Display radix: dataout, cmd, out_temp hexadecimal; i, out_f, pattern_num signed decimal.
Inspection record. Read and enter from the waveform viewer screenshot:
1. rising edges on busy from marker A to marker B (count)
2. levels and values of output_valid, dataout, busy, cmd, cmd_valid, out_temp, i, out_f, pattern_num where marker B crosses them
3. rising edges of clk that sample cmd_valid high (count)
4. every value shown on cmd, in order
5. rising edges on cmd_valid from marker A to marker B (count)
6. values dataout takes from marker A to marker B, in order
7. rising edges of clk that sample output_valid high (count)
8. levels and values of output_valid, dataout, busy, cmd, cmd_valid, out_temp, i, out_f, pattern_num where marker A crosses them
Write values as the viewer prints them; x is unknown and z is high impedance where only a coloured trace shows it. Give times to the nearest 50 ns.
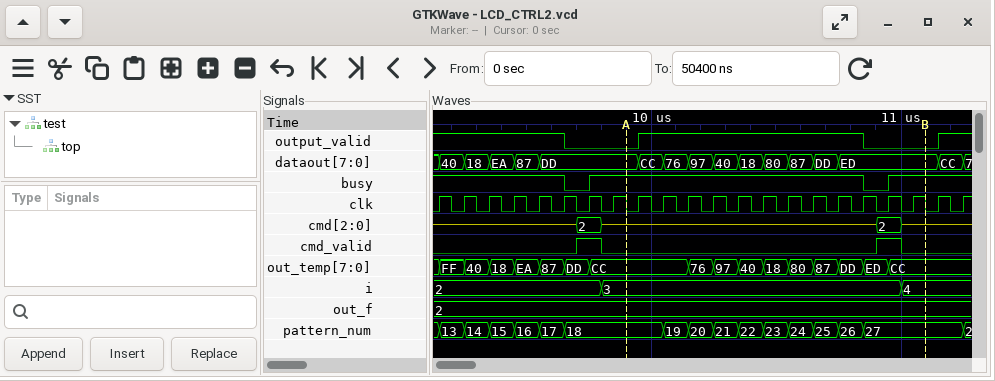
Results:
1
output_valid=0, dataout=ED, busy=1, cmd=z, cmd_valid=0, out_temp=CC, i=4, out_f=2, pattern_num=27
2
z, 2, z, 2, z
1
DD, CC, 76, 97, 40, 18, 80, 87, DD, ED
16
output_valid=0, dataout=DD, busy=1, cmd=z, cmd_valid=0, out_temp=CC, i=3, out_f=2, pattern_num=18
